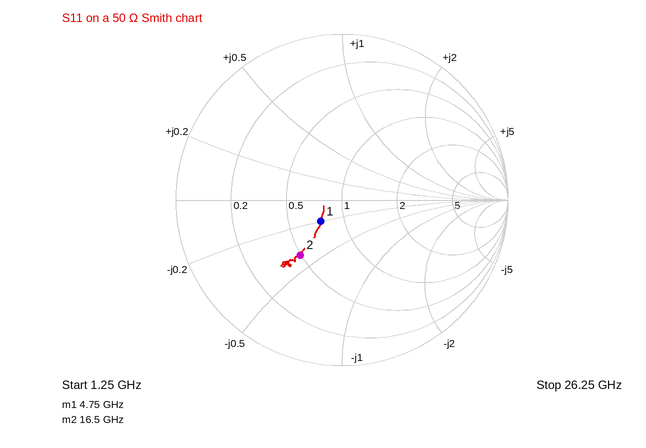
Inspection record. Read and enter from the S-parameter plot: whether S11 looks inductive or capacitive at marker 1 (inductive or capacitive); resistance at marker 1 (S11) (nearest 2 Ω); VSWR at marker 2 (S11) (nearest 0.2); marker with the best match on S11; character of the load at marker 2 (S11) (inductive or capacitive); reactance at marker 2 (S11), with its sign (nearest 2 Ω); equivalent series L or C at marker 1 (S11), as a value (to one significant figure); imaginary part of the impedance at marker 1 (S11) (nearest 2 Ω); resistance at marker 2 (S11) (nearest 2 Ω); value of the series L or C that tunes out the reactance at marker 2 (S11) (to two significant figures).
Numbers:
capacitive
38 Ω
2.4
marker 1
capacitive
-20 Ω
3 pF
-10 Ω
24 Ω
190 pH
